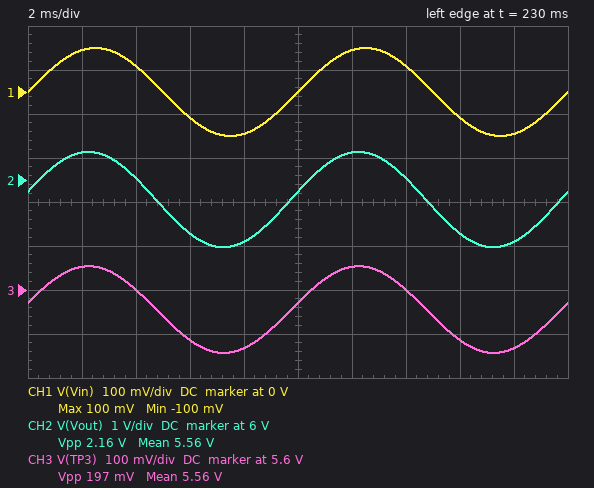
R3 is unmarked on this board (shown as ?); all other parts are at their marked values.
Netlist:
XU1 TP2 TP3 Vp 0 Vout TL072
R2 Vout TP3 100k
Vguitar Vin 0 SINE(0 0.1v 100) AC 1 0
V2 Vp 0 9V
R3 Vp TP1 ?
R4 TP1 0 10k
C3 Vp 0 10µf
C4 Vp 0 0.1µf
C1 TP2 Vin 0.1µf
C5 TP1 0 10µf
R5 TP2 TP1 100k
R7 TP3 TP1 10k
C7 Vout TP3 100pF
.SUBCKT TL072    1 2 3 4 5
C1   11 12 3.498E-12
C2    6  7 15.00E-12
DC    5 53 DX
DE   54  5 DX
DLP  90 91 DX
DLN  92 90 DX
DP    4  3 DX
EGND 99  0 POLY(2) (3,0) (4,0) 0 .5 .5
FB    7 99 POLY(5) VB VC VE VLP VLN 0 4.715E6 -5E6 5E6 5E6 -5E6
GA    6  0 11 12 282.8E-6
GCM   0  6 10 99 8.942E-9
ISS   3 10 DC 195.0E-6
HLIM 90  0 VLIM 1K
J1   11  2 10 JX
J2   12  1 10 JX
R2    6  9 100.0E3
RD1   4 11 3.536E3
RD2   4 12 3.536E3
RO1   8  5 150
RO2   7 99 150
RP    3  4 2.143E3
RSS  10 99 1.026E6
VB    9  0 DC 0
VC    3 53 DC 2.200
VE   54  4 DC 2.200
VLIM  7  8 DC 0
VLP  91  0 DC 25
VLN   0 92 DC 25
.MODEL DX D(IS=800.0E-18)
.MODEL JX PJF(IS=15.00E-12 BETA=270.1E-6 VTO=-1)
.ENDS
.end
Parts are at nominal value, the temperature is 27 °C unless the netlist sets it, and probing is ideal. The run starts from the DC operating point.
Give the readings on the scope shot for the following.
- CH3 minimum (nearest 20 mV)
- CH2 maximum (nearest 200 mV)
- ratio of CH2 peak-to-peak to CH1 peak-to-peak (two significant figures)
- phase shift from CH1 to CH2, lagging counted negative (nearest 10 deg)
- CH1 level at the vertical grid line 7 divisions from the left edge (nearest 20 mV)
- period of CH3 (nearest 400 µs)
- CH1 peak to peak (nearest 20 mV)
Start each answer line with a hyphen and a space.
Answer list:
- 5.46 V
- 6.6 V
- 11
- 10 deg
- 60 mV
- 10.0 ms
- 200 mV
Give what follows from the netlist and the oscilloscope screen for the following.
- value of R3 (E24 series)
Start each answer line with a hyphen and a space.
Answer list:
- 6.2 kΩ
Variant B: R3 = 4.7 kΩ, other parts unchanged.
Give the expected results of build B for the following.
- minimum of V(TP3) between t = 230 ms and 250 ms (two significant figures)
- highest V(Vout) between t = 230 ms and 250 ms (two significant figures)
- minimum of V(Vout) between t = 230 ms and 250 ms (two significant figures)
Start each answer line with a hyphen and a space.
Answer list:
- 6.0 V
- 7.2 V
- 5.0 V
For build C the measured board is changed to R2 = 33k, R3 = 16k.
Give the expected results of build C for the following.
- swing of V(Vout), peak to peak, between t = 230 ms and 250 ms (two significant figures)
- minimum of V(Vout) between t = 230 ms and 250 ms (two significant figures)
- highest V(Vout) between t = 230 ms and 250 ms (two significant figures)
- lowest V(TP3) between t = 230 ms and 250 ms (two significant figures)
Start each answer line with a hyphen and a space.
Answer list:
- 850 mV
- 3.0 V
- 3.9 V
- 3.4 V
